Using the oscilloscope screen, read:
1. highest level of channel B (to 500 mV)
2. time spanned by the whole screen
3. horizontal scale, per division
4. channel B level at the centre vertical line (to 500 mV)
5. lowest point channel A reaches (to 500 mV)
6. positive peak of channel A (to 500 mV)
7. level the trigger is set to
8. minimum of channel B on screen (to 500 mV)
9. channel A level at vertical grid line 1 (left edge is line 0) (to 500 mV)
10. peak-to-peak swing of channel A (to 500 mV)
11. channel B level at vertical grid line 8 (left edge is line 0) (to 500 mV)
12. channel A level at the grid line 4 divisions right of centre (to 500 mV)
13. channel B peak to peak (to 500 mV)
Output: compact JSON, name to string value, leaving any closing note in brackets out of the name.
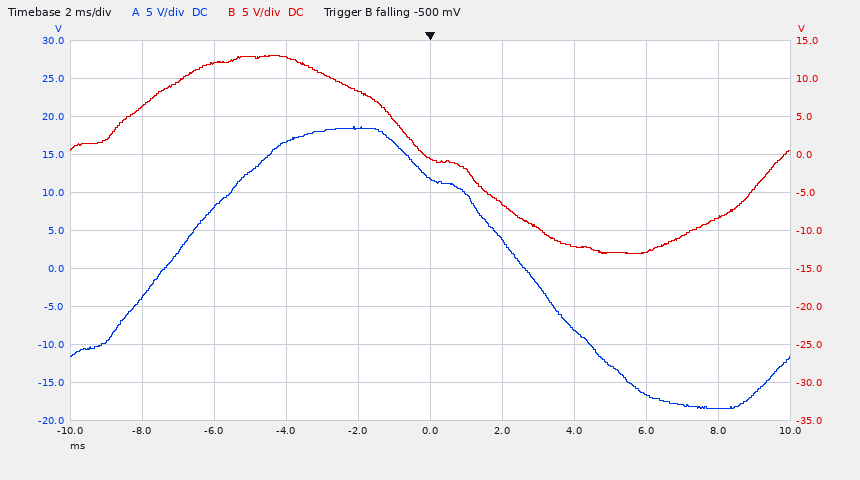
{"highest level of channel B": "13.0 V", "time spanned by the whole screen": "20 ms", "horizontal scale, per division": "2 ms", "channel B level at the centre vertical line": "-500 mV", "lowest point channel A reaches": "-18.5 V", "positive peak of channel A": "18.5 V", "level the trigger is set to": "-500 mV", "minimum of channel B on screen": "-13.0 V", "channel A level at vertical grid line 1 (left edge is line 0)": "-4.0 V", "peak-to-peak swing of channel A": "37.0 V", "channel B level at vertical grid line 8 (left edge is line 0)": "-13.0 V", "channel A level at the grid line 4 divisions right of centre": "-18.5 V", "channel B peak to peak": "26.0 V"}
